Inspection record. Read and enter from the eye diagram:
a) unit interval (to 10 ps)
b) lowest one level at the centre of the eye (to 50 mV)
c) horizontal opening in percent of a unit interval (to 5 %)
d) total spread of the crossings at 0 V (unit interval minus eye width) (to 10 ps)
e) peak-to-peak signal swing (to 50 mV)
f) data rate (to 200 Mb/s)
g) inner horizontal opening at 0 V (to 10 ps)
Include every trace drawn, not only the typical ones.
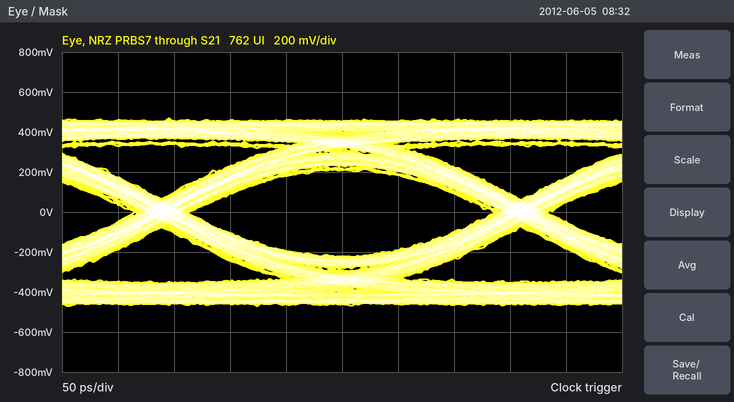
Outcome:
320 ps
200 mV
85 %
50 ps
950 mV
3.2 Gb/s
270 ps
